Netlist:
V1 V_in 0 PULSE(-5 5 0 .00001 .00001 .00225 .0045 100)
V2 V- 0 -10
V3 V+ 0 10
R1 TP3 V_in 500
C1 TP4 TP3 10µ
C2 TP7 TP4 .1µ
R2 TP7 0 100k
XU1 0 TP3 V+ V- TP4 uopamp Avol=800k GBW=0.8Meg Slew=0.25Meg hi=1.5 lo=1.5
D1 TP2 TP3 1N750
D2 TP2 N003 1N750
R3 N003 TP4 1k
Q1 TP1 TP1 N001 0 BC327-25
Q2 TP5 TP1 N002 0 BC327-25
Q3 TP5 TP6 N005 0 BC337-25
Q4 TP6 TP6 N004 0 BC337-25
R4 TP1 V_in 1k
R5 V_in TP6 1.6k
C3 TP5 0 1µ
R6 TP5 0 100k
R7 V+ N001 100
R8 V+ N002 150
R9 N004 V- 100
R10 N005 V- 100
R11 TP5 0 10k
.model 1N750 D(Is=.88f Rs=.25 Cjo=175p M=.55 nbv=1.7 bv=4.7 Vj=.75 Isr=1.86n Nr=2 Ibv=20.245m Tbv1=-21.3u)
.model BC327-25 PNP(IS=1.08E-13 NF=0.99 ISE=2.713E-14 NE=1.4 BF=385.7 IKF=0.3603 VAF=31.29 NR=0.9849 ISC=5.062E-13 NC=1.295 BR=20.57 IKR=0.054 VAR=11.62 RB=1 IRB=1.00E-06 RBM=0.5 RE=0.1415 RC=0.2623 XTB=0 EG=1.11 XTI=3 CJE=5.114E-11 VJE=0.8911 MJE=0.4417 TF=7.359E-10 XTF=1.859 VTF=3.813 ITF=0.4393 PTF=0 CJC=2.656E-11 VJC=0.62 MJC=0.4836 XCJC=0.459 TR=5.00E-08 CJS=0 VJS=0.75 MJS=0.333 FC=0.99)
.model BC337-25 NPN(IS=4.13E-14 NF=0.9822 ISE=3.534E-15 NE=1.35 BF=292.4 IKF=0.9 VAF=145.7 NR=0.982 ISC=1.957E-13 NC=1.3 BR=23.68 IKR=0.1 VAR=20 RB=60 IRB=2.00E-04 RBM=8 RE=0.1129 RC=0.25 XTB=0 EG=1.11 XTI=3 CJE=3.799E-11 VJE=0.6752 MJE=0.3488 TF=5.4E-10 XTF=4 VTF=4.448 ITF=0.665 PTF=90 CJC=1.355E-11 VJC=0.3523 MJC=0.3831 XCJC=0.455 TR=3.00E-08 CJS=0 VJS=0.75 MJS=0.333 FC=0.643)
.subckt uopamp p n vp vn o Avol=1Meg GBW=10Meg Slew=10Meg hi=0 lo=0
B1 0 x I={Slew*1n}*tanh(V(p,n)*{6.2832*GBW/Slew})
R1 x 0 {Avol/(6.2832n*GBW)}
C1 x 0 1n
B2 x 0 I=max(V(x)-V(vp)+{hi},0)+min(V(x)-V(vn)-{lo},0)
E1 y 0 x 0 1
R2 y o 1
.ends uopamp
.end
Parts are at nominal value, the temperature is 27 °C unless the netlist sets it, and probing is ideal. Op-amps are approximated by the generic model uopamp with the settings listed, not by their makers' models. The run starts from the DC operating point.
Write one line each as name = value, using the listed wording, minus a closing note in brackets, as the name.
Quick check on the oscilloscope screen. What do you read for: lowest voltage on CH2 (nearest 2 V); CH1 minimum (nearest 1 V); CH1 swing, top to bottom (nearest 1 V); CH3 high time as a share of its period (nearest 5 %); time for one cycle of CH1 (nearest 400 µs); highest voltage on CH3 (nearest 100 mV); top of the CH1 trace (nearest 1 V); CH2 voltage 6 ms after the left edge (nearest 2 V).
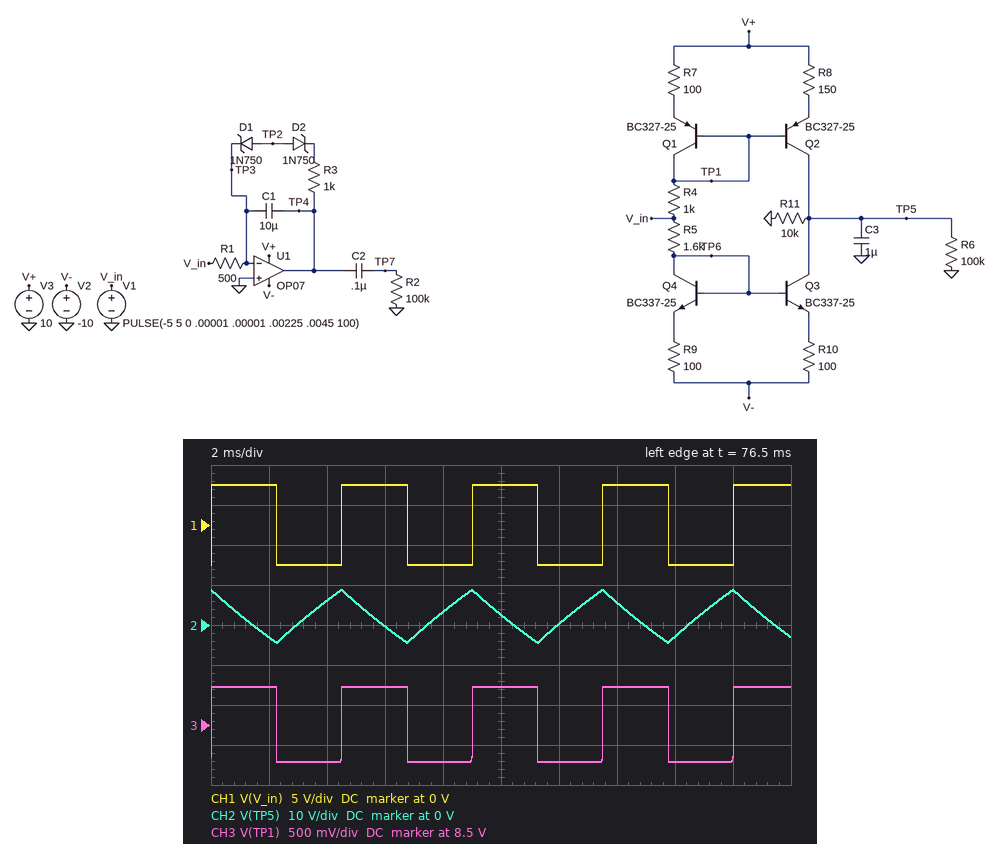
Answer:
lowest voltage on CH2 = -4 V
CH1 minimum = -5 V
CH1 swing, top to bottom = 10 V
CH3 high time as a share of its period = 50 %
time for one cycle of CH1 = 4.4 ms
highest voltage on CH3 = 9.0 V
top of the CH1 trace = 5 V
CH2 voltage 6 ms after the left edge = 0 V
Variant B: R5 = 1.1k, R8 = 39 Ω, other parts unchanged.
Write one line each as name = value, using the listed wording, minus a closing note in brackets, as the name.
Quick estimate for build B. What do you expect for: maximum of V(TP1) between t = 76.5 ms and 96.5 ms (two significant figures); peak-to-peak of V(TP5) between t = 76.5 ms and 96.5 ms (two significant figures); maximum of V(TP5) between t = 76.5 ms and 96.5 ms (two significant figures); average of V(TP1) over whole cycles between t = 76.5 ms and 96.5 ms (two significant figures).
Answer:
maximum of V(TP1) between t = 76.5 ms and 96.5 ms = 9.0 V
peak-to-peak of V(TP5) between t = 76.5 ms and 96.5 ms = 6.7 V
maximum of V(TP5) between t = 76.5 ms and 96.5 ms = 9.5 V
average of V(TP1) over whole cycles between t = 76.5 ms and 96.5 ms = 8.8 V
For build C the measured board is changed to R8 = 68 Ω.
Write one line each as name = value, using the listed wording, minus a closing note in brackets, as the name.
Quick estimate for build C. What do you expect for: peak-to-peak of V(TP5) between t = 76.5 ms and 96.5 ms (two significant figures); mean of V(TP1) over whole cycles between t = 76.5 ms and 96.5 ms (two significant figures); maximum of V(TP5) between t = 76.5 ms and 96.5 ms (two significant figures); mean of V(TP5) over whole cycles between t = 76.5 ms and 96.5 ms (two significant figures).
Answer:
peak-to-peak of V(TP5) between t = 76.5 ms and 96.5 ms = 7.4 V
mean of V(TP1) over whole cycles between t = 76.5 ms and 96.5 ms = 8.7 V
maximum of V(TP5) between t = 76.5 ms and 96.5 ms = 9.3 V
mean of V(TP5) over whole cycles between t = 76.5 ms and 96.5 ms = 7.0 V
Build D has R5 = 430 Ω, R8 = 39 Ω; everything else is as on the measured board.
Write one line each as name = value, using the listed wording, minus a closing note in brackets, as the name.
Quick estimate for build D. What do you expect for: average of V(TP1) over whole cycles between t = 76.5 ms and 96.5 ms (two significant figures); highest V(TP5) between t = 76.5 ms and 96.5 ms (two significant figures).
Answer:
average of V(TP1) over whole cycles between t = 76.5 ms and 96.5 ms = 8.7 V
highest V(TP5) between t = 76.5 ms and 96.5 ms = 9.4 V
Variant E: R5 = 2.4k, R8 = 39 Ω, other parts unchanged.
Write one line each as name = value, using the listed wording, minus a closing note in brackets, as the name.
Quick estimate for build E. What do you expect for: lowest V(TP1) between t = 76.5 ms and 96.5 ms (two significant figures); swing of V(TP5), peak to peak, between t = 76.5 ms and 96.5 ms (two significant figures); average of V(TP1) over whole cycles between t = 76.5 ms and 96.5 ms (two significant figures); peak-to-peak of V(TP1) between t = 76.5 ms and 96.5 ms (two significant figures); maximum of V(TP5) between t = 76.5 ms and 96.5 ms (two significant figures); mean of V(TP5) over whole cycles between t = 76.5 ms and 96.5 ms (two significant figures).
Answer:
lowest V(TP1) between t = 76.5 ms and 96.5 ms = 8.8 V
swing of V(TP5), peak to peak, between t = 76.5 ms and 96.5 ms = 140 mV
average of V(TP1) over whole cycles between t = 76.5 ms and 96.5 ms = 8.9 V
peak-to-peak of V(TP1) between t = 76.5 ms and 96.5 ms = 210 mV
maximum of V(TP5) between t = 76.5 ms and 96.5 ms = 9.7 V
mean of V(TP5) over whole cycles between t = 76.5 ms and 96.5 ms = 9.6 V
